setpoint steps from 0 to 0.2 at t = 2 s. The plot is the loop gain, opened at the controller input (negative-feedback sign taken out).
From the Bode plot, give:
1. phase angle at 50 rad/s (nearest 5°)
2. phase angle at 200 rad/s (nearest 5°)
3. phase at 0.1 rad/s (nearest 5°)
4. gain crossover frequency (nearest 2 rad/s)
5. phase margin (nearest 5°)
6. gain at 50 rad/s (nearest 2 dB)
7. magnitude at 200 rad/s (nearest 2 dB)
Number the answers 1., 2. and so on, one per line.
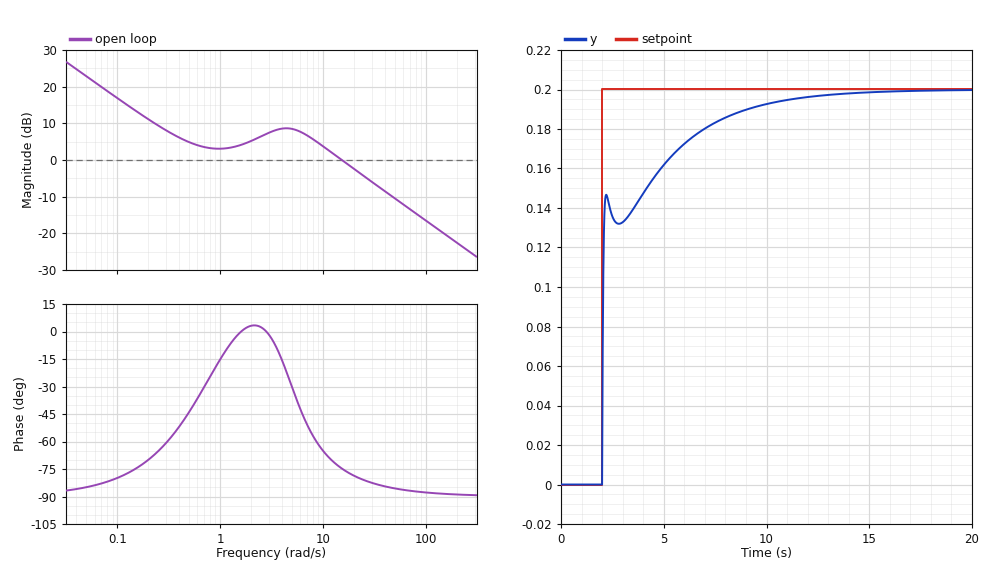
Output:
1. -85°
2. -90°
3. -80°
4. 16 rad/s
5. 105°
6. -10 dB
7. -22 dB
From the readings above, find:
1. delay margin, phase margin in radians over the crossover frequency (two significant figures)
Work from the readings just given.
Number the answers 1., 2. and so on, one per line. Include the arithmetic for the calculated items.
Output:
1. 105 × π / 180 / 16 = 0.11 s
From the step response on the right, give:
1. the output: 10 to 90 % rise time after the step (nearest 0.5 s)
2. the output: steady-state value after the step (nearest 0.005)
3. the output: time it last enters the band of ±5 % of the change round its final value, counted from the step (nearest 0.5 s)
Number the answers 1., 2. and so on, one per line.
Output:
1. 5.0 s
2. 0.200
3. 7.0 s
